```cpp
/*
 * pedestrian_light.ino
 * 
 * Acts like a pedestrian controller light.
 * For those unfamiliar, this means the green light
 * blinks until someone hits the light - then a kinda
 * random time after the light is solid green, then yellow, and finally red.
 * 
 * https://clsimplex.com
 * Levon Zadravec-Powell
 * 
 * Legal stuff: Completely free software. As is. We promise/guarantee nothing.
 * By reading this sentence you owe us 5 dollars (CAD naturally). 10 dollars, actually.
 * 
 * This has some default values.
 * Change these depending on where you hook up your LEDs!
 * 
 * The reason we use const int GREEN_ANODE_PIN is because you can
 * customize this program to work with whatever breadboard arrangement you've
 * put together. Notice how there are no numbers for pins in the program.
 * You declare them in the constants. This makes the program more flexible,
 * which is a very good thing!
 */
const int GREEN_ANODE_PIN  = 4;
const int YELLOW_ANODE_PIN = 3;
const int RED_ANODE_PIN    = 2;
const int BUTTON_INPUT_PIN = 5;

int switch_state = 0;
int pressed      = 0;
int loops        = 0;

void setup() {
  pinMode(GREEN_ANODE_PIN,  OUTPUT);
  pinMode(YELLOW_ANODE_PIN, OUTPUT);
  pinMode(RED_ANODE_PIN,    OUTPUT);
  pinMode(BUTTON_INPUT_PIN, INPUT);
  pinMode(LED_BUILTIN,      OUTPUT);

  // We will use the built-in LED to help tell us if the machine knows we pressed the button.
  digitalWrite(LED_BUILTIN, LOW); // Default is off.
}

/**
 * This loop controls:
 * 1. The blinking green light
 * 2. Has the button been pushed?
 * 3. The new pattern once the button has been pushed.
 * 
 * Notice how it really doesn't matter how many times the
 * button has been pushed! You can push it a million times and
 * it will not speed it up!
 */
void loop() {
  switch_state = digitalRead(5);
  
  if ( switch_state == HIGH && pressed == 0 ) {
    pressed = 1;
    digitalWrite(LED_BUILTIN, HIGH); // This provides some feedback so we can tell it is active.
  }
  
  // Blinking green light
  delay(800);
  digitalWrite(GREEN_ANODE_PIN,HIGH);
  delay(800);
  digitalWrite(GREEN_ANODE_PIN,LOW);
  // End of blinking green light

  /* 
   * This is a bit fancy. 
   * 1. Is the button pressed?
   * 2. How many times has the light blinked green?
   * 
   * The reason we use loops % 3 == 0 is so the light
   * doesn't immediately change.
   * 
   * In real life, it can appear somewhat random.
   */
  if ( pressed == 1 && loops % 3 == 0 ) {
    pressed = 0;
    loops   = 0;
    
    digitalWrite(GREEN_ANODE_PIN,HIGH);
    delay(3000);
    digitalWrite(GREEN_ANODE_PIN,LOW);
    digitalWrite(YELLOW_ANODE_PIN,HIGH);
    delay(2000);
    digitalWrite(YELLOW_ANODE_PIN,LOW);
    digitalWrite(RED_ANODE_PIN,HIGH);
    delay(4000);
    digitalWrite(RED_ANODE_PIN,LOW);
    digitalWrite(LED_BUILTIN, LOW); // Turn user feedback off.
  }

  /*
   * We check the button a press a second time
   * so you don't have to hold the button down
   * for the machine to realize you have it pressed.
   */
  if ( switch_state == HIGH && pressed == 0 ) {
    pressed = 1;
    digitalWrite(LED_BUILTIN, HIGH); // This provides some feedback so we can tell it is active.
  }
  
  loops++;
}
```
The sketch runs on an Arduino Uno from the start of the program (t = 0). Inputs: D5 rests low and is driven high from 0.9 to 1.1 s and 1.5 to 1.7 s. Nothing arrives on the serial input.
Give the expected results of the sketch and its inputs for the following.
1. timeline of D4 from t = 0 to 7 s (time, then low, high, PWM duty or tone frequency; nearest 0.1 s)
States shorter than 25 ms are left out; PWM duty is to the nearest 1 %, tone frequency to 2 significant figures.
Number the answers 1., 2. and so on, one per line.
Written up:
1. 0 s low; 0.8 s high; 1.6 s low; 2.4 s high; 3.2 s low; 4 s high; 4.8 s low; 5.6 s high
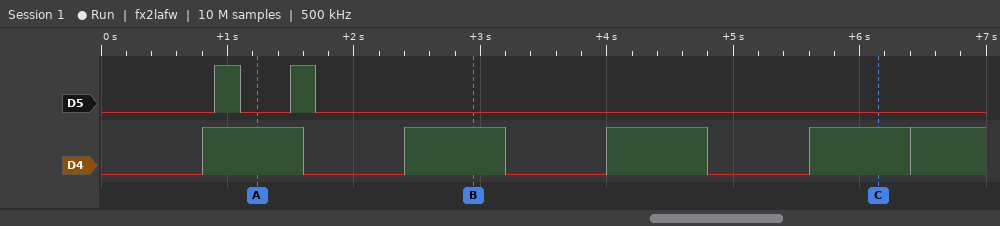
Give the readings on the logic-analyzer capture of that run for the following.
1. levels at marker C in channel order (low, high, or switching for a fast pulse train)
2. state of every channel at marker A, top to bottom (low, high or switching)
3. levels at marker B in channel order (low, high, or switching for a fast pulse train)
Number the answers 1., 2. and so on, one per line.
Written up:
1. D5 low, D4 high
2. D5 low, D4 high
3. D5 low, D4 high
